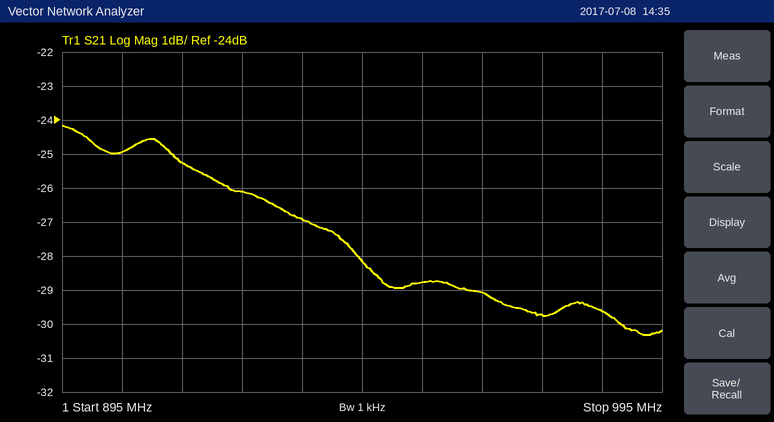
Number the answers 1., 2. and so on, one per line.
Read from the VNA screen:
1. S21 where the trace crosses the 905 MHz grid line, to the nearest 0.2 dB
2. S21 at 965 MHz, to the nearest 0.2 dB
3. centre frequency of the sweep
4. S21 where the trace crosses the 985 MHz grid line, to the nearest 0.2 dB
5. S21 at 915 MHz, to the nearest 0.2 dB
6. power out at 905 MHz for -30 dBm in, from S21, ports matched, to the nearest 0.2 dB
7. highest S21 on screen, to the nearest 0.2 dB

1. -25.0 dB
2. -29.0 dB
3. 945 MHz
4. -29.6 dB
5. -25.2 dB
6. -55.0 dBm
7. -24.2 dB
